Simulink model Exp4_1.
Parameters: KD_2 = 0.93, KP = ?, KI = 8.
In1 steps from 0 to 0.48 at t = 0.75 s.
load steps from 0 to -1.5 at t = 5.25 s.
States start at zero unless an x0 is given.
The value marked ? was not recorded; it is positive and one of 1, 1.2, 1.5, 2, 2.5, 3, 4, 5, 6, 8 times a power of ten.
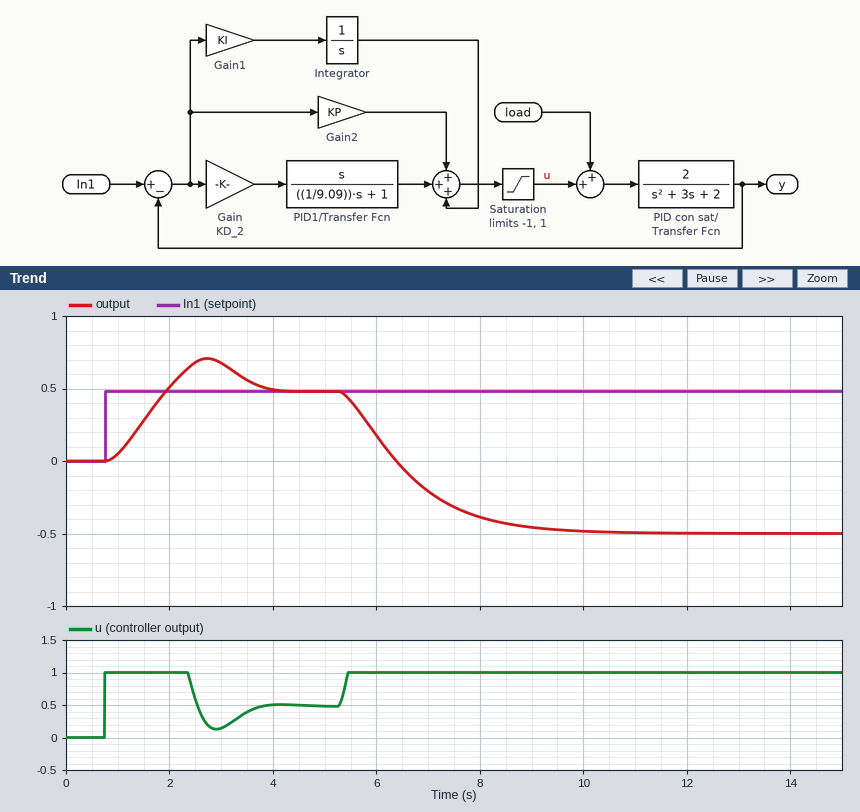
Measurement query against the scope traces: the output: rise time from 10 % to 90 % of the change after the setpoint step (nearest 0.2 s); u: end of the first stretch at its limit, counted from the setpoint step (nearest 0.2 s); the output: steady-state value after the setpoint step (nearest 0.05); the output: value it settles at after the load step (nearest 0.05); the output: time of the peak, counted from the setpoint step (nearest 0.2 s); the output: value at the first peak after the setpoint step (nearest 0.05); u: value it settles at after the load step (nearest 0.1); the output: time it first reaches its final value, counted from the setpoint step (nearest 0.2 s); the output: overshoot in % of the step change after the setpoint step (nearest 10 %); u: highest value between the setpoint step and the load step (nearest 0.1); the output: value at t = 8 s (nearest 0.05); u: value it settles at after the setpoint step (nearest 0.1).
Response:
0.8 s
1.6 s
0.50
-0.50
2.0 s
0.70
1.0
1.2 s
50 %
1.0
-0.40
0.5
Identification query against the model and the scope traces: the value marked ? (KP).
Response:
6
